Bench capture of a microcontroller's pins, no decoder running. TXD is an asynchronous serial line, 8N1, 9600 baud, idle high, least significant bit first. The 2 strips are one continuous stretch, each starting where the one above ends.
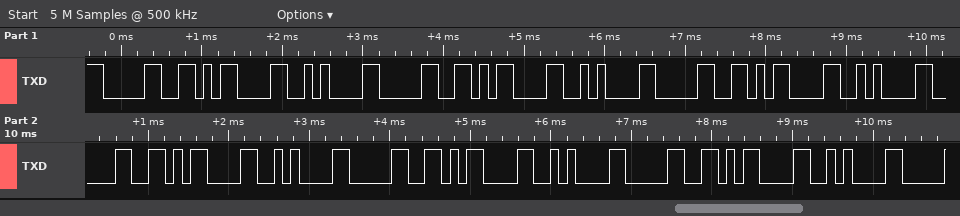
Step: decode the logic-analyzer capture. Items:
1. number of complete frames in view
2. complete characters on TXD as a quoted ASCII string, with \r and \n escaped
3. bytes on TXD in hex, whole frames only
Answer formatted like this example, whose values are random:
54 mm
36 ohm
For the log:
18
"0\r\n0\r\n0\r\n0\r\n0\r\n0\r\n"
30 0D 0A 30 0D 0A 30 0D 0A 30 0D 0A 30 0D 0A 30 0D 0A
